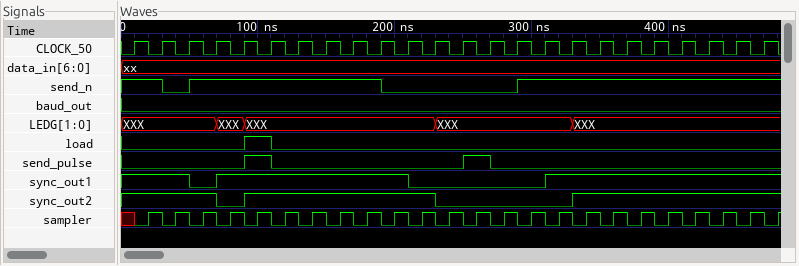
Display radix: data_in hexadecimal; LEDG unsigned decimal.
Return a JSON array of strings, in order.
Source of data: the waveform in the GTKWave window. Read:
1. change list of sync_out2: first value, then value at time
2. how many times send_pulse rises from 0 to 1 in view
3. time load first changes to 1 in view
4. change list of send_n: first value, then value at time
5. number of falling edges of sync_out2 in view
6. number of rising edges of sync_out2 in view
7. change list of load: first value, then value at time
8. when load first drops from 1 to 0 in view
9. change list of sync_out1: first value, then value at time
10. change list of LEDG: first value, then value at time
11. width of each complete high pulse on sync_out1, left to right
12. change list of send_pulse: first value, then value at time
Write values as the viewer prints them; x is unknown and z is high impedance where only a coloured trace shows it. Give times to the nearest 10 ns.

["1, 0 at 70 ns, 1 at 90 ns, 0 at 230 ns, 1 at 330 ns", "2", "90 ns", "1, 0 at 30 ns, 1 at 50 ns, 0 at 190 ns, 1 at 290 ns", "2", "2", "0, 1 at 90 ns, 0 at 110 ns", "110 ns", "1, 0 at 50 ns, 1 at 70 ns, 0 at 210 ns, 1 at 310 ns", "XXX, XXX at 70 ns, XXX at 90 ns, XXX at 230 ns, XXX at 330 ns", "140 ns", "0, 1 at 90 ns, 0 at 110 ns, 1 at 250 ns, 0 at 270 ns"]
